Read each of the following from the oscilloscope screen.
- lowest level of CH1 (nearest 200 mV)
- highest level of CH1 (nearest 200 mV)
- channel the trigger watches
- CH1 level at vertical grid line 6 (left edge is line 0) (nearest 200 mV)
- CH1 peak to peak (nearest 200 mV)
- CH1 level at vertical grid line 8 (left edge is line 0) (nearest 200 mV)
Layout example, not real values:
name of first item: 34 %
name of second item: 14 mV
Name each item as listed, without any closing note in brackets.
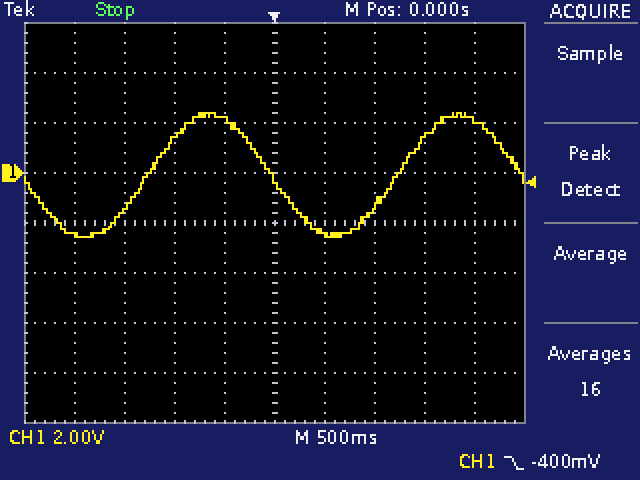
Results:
lowest level of CH1: -2.6 V
highest level of CH1: 2.4 V
channel the trigger watches: CH1
CH1 level at vertical grid line 6 (left edge is line 0): -2.4 V
CH1 peak to peak: 5.0 V
CH1 level at vertical grid line 8 (left edge is line 0): 1.4 V
